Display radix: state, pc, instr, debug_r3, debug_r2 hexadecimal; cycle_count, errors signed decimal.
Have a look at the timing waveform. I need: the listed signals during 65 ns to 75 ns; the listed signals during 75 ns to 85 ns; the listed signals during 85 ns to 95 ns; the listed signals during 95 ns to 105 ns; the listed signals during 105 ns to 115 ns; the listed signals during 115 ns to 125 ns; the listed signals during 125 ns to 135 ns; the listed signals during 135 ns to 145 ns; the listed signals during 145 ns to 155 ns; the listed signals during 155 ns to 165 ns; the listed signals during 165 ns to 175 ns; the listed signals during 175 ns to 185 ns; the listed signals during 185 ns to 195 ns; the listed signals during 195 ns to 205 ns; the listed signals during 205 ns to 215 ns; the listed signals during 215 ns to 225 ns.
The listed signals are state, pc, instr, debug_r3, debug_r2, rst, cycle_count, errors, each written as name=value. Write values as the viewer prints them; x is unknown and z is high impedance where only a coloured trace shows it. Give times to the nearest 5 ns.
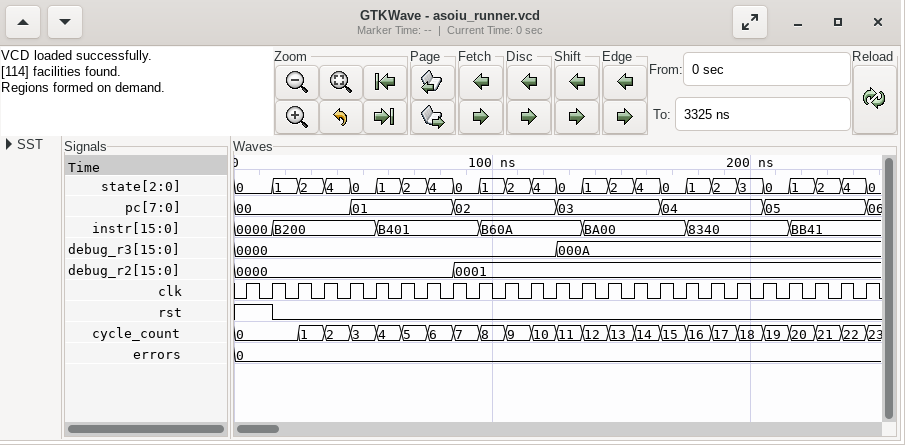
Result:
state=2, pc=01, instr=B401, debug_r3=0000, debug_r2=0000, rst=0, cycle_count=5, errors=0
state=4, pc=01, instr=B401, debug_r3=0000, debug_r2=0000, rst=0, cycle_count=6, errors=0
state=0, pc=02, instr=B401, debug_r3=0000, debug_r2=0001, rst=0, cycle_count=7, errors=0
state=1, pc=02, instr=B60A, debug_r3=0000, debug_r2=0001, rst=0, cycle_count=8, errors=0
state=2, pc=02, instr=B60A, debug_r3=0000, debug_r2=0001, rst=0, cycle_count=9, errors=0
state=4, pc=02, instr=B60A, debug_r3=0000, debug_r2=0001, rst=0, cycle_count=10, errors=0
state=0, pc=03, instr=B60A, debug_r3=000A, debug_r2=0001, rst=0, cycle_count=11, errors=0
state=1, pc=03, instr=BA00, debug_r3=000A, debug_r2=0001, rst=0, cycle_count=12, errors=0
state=2, pc=03, instr=BA00, debug_r3=000A, debug_r2=0001, rst=0, cycle_count=13, errors=0
state=4, pc=03, instr=BA00, debug_r3=000A, debug_r2=0001, rst=0, cycle_count=14, errors=0
state=0, pc=04, instr=BA00, debug_r3=000A, debug_r2=0001, rst=0, cycle_count=15, errors=0
state=1, pc=04, instr=8340, debug_r3=000A, debug_r2=0001, rst=0, cycle_count=16, errors=0
state=2, pc=04, instr=8340, debug_r3=000A, debug_r2=0001, rst=0, cycle_count=17, errors=0
state=3, pc=04, instr=8340, debug_r3=000A, debug_r2=0001, rst=0, cycle_count=18, errors=0
state=0, pc=05, instr=8340, debug_r3=000A, debug_r2=0001, rst=0, cycle_count=19, errors=0
state=1, pc=05, instr=BB41, debug_r3=000A, debug_r2=0001, rst=0, cycle_count=20, errors=0
